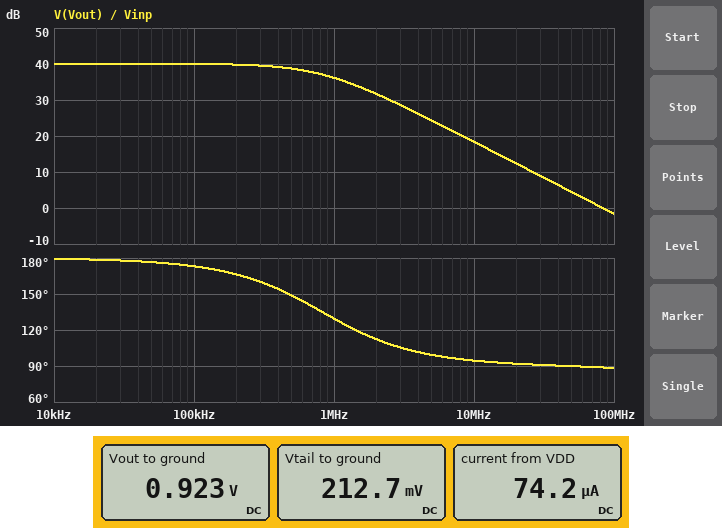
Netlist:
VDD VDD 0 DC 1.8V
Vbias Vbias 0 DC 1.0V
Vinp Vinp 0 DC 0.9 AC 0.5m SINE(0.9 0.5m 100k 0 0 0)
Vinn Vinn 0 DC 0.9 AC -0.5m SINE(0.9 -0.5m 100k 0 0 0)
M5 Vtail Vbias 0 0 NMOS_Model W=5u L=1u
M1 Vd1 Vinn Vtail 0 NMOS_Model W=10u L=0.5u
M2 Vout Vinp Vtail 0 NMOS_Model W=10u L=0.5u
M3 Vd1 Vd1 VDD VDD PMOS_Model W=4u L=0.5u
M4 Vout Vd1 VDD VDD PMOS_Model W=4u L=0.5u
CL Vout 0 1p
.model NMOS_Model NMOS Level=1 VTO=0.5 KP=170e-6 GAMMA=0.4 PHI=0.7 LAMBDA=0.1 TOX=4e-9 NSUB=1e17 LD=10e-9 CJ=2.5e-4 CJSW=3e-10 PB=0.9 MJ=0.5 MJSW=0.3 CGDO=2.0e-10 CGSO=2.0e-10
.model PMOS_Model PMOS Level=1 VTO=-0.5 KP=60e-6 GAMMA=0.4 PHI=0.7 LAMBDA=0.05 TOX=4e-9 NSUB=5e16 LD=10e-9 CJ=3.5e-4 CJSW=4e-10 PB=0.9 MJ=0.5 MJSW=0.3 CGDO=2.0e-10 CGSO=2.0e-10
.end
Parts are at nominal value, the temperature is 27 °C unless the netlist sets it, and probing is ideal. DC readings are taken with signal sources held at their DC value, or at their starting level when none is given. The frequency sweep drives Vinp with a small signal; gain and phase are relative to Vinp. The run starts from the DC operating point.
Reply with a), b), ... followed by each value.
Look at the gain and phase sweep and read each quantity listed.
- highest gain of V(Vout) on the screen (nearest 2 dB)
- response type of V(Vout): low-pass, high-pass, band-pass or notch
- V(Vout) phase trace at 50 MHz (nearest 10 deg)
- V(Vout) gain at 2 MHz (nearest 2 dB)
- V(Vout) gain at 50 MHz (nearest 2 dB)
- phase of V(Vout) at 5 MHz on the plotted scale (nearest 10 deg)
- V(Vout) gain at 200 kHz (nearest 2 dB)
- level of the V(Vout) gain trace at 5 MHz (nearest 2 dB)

a) 40 dB
b) low-pass
c) 90 deg
d) 32 dB
e) 4 dB
f) 100 deg
g) 40 dB
h) 24 dB
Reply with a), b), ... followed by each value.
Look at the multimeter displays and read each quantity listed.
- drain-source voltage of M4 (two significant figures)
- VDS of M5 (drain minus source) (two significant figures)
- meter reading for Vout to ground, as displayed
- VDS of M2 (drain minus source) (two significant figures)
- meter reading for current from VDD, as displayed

a) -880 mV
b) 210 mV
c) 0.923 V
d) 710 mV
e) 74.2 µA
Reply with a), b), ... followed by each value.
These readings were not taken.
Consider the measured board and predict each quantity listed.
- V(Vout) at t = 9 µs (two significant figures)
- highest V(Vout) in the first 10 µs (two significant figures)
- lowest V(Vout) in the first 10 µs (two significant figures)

a) 990 mV
b) 1.0 V
c) 820 mV
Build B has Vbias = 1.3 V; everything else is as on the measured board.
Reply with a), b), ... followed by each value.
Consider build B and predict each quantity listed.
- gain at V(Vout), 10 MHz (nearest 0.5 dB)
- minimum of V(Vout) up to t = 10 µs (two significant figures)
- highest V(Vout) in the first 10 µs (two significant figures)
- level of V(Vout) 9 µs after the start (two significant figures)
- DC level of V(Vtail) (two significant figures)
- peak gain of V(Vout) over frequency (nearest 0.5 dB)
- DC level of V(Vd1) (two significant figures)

a) 20.0 dB
b) 750 mV
c) 910 mV
d) 880 mV
e) 180 mV
f) 38.0 dB
g) 830 mV
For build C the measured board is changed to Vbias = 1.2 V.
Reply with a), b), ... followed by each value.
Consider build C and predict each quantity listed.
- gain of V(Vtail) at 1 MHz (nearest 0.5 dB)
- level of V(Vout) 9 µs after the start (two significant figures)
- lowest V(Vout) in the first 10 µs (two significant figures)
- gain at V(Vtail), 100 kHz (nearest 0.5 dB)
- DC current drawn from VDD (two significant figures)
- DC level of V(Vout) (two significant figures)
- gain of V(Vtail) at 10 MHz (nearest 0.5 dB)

a) -13.0 dB
b) 910 mV
c) 770 mV
d) -19.0 dB
e) 100 µA
f) 860 mV
g) -10.0 dB
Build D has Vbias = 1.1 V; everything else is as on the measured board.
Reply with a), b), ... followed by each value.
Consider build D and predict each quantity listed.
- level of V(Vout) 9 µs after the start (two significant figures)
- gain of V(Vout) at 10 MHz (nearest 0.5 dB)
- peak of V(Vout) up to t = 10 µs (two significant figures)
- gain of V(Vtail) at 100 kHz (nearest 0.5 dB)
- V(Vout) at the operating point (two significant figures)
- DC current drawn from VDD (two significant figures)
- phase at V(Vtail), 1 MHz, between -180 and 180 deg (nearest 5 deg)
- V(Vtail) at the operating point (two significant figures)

a) 950 mV
b) 19.0 dB
c) 980 mV
d) -18.5 dB
e) 890 mV
f) 89 µA
g) 25 deg
h) 200 mV
